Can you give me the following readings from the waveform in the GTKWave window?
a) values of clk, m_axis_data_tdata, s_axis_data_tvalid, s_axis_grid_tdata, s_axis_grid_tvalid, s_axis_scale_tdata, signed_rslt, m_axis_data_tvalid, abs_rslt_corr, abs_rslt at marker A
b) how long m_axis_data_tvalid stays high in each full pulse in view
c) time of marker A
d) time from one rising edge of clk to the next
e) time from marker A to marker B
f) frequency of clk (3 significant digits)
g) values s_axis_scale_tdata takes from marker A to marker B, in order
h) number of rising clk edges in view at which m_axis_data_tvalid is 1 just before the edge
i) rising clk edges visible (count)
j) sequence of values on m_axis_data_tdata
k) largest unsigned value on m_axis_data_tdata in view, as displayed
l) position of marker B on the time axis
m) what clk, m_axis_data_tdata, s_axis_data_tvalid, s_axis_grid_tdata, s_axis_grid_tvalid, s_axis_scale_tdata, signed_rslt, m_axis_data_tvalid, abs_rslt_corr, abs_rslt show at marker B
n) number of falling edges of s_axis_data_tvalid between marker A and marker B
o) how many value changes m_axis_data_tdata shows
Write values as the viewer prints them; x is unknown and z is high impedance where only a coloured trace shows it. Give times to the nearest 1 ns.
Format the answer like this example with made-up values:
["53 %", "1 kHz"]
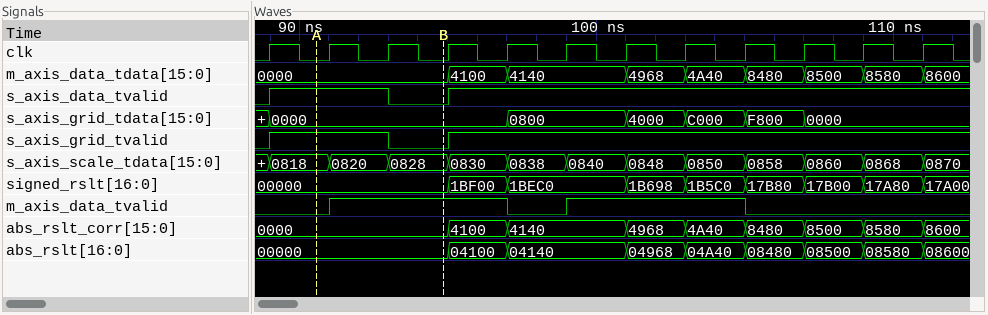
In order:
["clk=0, m_axis_data_tdata=0000, s_axis_data_tvalid=1, s_axis_grid_tdata=0000, s_axis_grid_tvalid=1, s_axis_scale_tdata=0818, signed_rslt=00000, m_axis_data_tvalid=0, abs_rslt_corr=0000, abs_rslt=00000", "6 ns, 6 ns", "91 ns", "2 ns", "4 ns", "500 MHz", "0818, 0820, 0828", "6", "12", "0000, 4100, 4140, 4968, 4A40, 8480, 8500, 8580, 8600", "8600", "95 ns", "clk=0, m_axis_data_tdata=0000, s_axis_data_tvalid=0, s_axis_grid_tdata=0000, s_axis_grid_tvalid=0, s_axis_scale_tdata=0828, signed_rslt=00000, m_axis_data_tvalid=1, abs_rslt_corr=0000, abs_rslt=00000", "1", "8"]
